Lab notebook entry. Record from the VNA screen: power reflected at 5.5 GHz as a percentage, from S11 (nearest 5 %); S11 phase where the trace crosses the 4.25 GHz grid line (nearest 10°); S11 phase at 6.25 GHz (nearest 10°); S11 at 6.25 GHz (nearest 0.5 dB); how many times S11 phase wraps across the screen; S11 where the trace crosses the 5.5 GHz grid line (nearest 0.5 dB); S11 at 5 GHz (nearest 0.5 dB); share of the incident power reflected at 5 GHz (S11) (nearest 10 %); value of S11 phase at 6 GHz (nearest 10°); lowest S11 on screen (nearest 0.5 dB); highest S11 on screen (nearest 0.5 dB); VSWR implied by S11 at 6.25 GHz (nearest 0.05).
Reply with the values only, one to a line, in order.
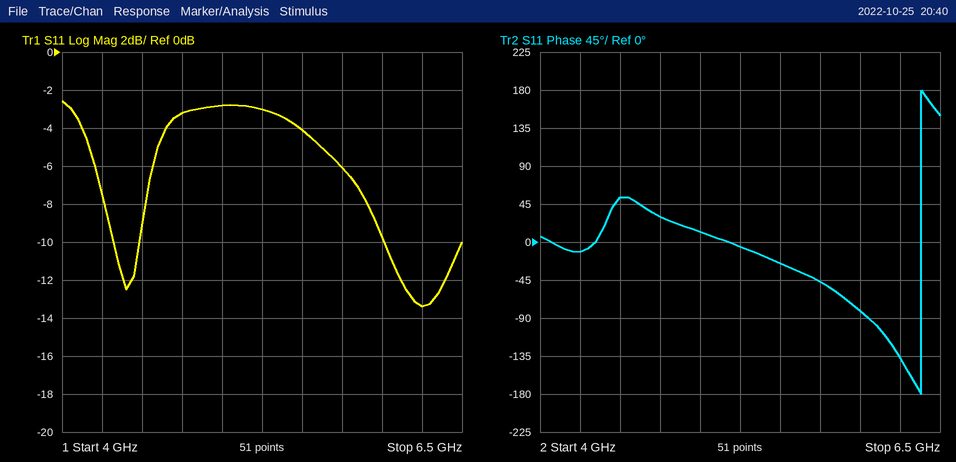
40 %
-10°
-140°
-13.5 dB
1
-4.0 dB
-3.0 dB
50 %
-80°
-13.5 dB
-2.5 dB
1.55
